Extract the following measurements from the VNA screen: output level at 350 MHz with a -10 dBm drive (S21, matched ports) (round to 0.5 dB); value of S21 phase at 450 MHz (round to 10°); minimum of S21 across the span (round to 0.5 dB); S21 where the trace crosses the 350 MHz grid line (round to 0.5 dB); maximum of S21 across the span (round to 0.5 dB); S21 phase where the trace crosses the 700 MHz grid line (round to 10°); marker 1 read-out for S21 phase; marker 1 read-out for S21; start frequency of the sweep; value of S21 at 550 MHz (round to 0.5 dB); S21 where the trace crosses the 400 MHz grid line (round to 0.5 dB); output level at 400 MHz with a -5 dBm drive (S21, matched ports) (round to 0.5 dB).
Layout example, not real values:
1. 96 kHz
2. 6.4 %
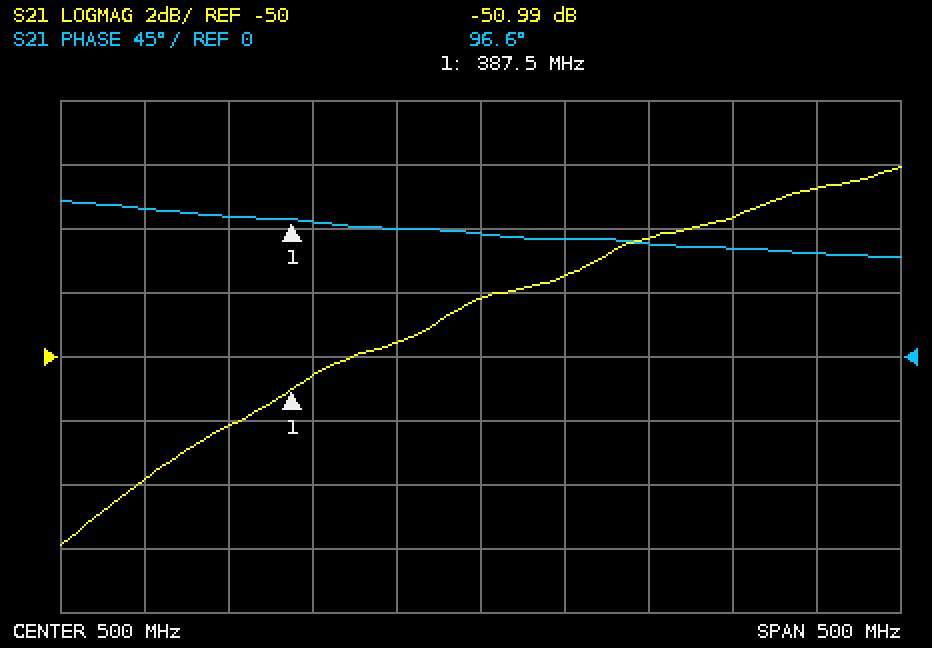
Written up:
1. -62.0 dBm
2. 90°
3. -56.0 dB
4. -52.0 dB
5. -44.0 dB
6. 70°
7. 96.6°
8. -50.99 dB
9. 250 MHz
10. -47.5 dB
11. -50.5 dB
12. -55.5 dBm
